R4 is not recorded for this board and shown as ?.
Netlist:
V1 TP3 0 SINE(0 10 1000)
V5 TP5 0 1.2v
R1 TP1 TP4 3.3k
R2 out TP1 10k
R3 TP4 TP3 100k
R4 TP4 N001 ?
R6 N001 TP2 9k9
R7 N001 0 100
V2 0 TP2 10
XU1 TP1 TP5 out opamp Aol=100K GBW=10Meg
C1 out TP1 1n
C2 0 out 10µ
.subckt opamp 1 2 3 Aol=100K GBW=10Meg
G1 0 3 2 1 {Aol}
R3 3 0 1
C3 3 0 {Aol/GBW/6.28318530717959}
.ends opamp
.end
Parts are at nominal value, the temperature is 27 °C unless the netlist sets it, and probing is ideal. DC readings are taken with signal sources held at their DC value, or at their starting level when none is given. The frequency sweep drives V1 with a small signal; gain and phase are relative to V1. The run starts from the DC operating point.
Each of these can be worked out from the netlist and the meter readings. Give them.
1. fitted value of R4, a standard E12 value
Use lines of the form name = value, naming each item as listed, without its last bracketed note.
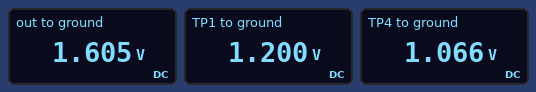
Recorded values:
fitted value of R4, a standard E12 value = 39 kΩ
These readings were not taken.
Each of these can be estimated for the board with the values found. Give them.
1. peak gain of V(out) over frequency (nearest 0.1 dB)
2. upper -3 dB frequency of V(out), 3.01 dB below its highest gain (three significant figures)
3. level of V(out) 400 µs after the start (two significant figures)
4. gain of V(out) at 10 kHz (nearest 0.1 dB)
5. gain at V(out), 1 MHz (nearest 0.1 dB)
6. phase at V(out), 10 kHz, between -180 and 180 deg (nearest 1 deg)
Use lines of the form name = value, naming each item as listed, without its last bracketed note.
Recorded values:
peak gain of V(out) over frequency = -21.0 dB
upper -3 dB frequency of V(out), 3.01 dB below its highest gain = 15.9 kHz
level of V(out) 400 µs after the start = 1.0 V
gain of V(out) at 10 kHz = -22.4 dB
gain at V(out), 1 MHz = -57.0 dB
phase at V(out), 10 kHz, between -180 and 180 deg = 148 deg
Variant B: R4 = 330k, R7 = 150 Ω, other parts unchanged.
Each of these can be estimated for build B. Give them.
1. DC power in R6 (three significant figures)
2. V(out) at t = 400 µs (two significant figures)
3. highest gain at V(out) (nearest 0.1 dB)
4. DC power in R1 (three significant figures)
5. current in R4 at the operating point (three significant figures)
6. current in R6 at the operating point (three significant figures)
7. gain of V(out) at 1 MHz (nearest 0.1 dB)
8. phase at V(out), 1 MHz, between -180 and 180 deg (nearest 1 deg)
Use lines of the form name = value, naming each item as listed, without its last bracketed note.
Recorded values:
DC power in R6 = 9.80 mW
V(out) at t = 400 µs = 740 mV
highest gain at V(out) = -20.4 dB
DC power in R1 = 785 nW
current in R4 at the operating point = 3.93 µA
current in R6 at the operating point = 995 µA
gain of V(out) at 1 MHz = -56.4 dB
phase at V(out), 1 MHz, between -180 and 180 deg = 85 deg
